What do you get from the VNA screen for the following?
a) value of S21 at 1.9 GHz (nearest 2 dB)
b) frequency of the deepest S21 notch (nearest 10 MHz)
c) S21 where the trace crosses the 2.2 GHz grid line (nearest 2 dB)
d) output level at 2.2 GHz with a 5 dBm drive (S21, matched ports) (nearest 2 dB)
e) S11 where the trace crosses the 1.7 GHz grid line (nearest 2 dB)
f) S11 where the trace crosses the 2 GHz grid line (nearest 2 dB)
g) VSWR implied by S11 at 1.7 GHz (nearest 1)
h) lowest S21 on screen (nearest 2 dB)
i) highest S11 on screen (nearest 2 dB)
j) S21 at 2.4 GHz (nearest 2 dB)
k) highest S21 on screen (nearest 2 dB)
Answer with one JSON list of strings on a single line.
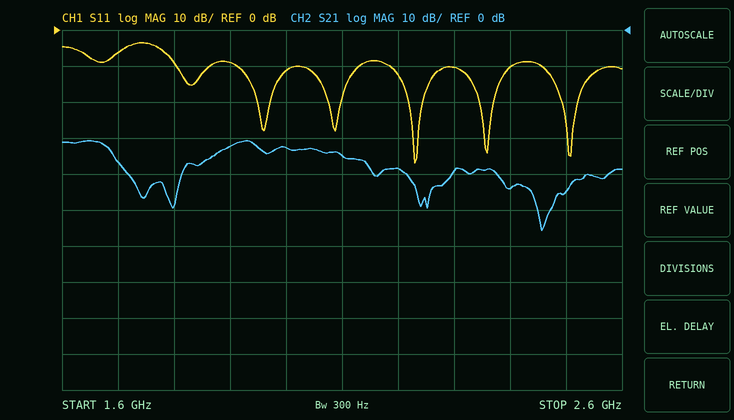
["-32 dB", "2.46 GHz", "-38 dB", "-34 dBm", "-6 dB", "-12 dB", "3", "-56 dB", "-4 dB", "-44 dB", "-30 dB"]
